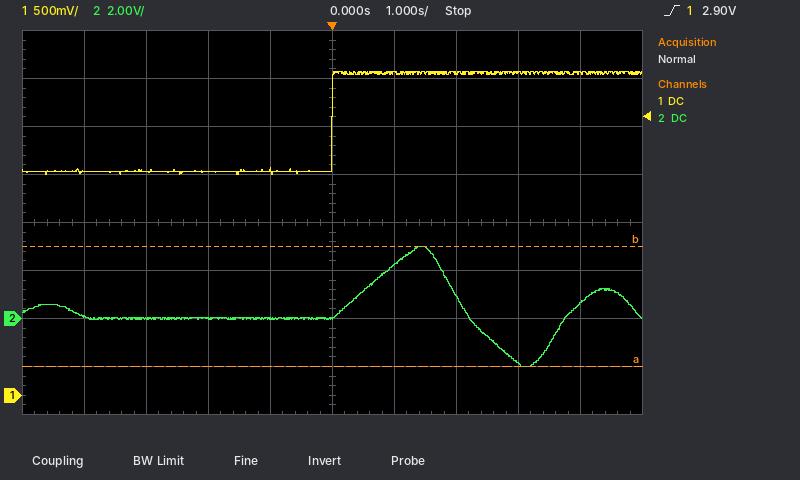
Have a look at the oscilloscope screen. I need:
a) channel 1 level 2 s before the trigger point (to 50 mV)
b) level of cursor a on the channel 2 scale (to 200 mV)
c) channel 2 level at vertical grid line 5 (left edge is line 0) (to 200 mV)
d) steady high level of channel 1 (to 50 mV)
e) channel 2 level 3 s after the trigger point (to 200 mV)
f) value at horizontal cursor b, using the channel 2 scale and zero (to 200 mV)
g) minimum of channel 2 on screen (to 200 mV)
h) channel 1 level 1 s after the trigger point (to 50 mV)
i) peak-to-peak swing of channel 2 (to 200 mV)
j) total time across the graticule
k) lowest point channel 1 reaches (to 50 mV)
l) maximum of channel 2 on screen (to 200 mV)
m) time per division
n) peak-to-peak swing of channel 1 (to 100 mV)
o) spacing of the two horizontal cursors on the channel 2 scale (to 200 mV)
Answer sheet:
2.35 V
-2.0 V
0.0 V
3.35 V
-1.8 V
3.0 V
-2.0 V
3.35 V
5.0 V
10 s
2.30 V
3.0 V
1 s
1.10 V
5.0 V
